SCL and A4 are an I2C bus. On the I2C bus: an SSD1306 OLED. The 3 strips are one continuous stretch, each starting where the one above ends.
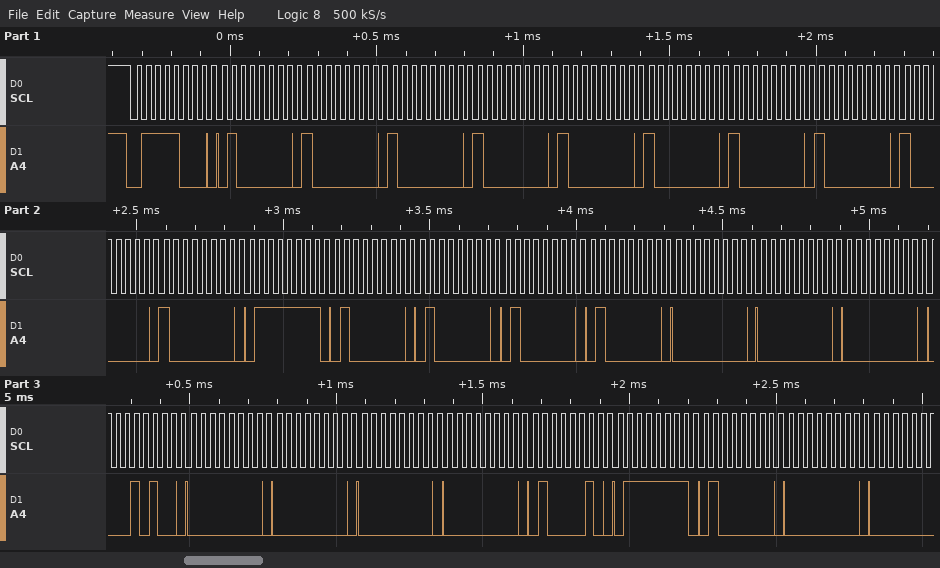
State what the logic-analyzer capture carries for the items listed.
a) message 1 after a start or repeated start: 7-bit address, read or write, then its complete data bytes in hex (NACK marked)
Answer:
0x3C write: 40 80 80 80 80 80 80 80 80 80 7F 40 40 40 40 00 00 00 14 00 00 00 00 42 7F 40 00
